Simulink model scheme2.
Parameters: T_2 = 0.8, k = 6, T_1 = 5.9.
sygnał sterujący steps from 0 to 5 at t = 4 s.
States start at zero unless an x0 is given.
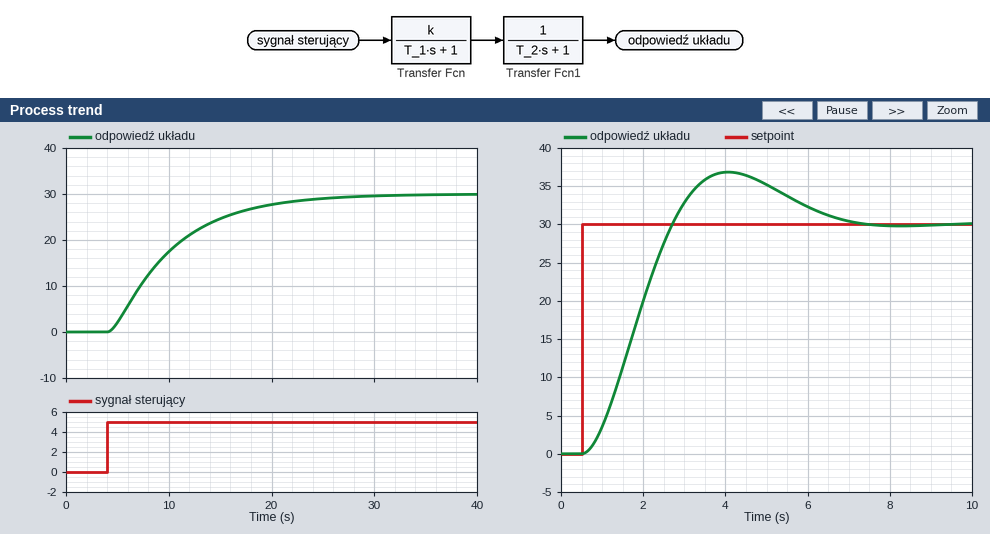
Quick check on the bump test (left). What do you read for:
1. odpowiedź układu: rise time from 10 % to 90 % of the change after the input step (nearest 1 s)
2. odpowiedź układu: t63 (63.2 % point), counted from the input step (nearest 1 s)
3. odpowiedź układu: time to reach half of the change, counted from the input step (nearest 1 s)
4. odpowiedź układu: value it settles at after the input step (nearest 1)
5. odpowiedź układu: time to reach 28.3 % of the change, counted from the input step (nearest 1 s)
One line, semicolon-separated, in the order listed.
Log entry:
13 s; 7 s; 5 s; 30; 3 s
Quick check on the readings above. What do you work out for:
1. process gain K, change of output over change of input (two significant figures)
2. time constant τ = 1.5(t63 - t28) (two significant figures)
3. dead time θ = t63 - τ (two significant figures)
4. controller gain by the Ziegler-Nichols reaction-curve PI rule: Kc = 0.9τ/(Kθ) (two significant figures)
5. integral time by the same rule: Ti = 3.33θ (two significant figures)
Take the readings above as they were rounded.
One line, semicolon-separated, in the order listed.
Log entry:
6.0; 6.0 s; 1.0 s; 0.90; 3.3 s
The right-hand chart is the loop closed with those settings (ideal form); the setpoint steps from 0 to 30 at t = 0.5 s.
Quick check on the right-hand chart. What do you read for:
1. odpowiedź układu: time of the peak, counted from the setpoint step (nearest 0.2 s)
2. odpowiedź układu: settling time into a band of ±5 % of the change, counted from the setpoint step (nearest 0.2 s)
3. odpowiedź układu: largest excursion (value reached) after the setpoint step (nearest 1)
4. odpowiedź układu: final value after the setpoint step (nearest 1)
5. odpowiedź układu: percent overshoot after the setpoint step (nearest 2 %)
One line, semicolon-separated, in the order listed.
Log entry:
3.6 s; 5.8 s; 37; 30; 22 %
